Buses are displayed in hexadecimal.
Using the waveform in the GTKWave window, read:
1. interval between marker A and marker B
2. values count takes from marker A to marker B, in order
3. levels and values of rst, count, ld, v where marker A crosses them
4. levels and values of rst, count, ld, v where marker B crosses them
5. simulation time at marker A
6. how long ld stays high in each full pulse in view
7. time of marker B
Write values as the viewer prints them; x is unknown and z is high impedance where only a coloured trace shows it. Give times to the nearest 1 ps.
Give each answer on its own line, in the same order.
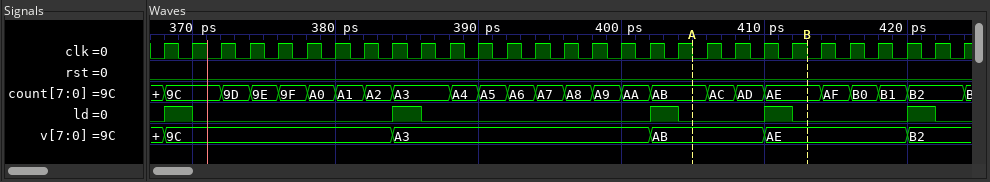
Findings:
8 ps
AB, AC, AD, AE
rst=0, count=AB, ld=0, v=AB
rst=0, count=AE, ld=0, v=AE
405 ps
2 ps, 2 ps, 2 ps, 2 ps, 2 ps
413 ps
